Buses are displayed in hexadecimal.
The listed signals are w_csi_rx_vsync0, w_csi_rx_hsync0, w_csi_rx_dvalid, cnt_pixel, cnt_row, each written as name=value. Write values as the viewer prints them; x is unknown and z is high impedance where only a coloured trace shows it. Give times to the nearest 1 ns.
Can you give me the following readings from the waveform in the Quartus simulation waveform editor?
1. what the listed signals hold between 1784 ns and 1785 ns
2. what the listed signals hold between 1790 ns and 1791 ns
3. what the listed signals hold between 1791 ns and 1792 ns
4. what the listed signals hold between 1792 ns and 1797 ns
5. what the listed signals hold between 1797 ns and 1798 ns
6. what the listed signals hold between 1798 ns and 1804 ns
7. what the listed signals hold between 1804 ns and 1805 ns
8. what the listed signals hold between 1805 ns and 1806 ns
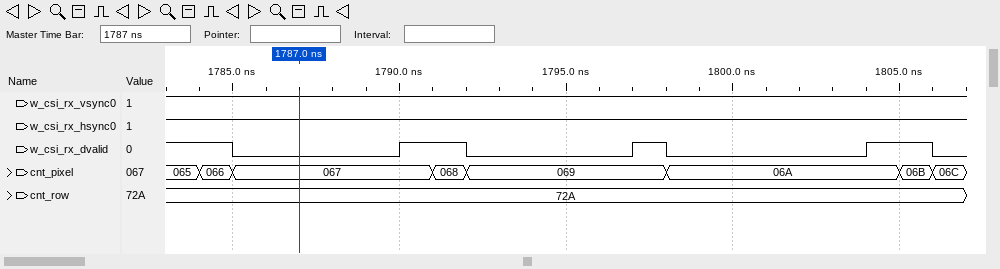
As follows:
w_csi_rx_vsync0=1, w_csi_rx_hsync0=1, w_csi_rx_dvalid=1, cnt_pixel=066, cnt_row=72A
w_csi_rx_vsync0=1, w_csi_rx_hsync0=1, w_csi_rx_dvalid=1, cnt_pixel=067, cnt_row=72A
w_csi_rx_vsync0=1, w_csi_rx_hsync0=1, w_csi_rx_dvalid=1, cnt_pixel=068, cnt_row=72A
w_csi_rx_vsync0=1, w_csi_rx_hsync0=1, w_csi_rx_dvalid=0, cnt_pixel=069, cnt_row=72A
w_csi_rx_vsync0=1, w_csi_rx_hsync0=1, w_csi_rx_dvalid=1, cnt_pixel=069, cnt_row=72A
w_csi_rx_vsync0=1, w_csi_rx_hsync0=1, w_csi_rx_dvalid=0, cnt_pixel=06A, cnt_row=72A
w_csi_rx_vsync0=1, w_csi_rx_hsync0=1, w_csi_rx_dvalid=1, cnt_pixel=06A, cnt_row=72A
w_csi_rx_vsync0=1, w_csi_rx_hsync0=1, w_csi_rx_dvalid=1, cnt_pixel=06B, cnt_row=72A
